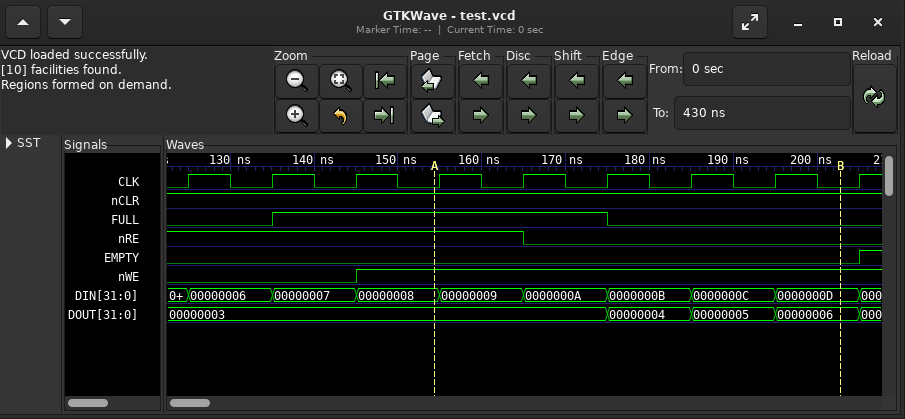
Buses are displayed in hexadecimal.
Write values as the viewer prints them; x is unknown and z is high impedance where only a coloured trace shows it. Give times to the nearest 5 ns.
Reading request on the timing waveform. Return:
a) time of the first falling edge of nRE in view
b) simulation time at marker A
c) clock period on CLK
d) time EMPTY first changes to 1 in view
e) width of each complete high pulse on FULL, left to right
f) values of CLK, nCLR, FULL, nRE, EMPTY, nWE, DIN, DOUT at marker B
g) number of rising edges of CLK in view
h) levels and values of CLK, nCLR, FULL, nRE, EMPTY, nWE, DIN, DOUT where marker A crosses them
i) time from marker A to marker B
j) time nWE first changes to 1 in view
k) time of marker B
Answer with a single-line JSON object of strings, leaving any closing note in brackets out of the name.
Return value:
{"time of the first falling edge of nRE in view": "165 ns", "simulation time at marker A": "155 ns", "clock period on CLK": "10 ns", "time EMPTY first changes to 1 in view": "205 ns", "width of each complete high pulse on FULL, left to right": "40 ns", "values of CLK, nCLR, FULL, nRE, EMPTY, nWE, DIN, DOUT at marker B": "CLK=0, nCLR=1, FULL=0, nRE=0, EMPTY=0, nWE=1, DIN=0000000D, DOUT=00000006", "number of rising edges of CLK in view": "9", "levels and values of CLK, nCLR, FULL, nRE, EMPTY, nWE, DIN, DOUT where marker A crosses them": "CLK=0, nCLR=1, FULL=1, nRE=1, EMPTY=0, nWE=1, DIN=00000008, DOUT=00000003", "time from marker A to marker B": "50 ns", "time nWE first changes to 1 in view": "145 ns", "time of marker B": "205 ns"}
